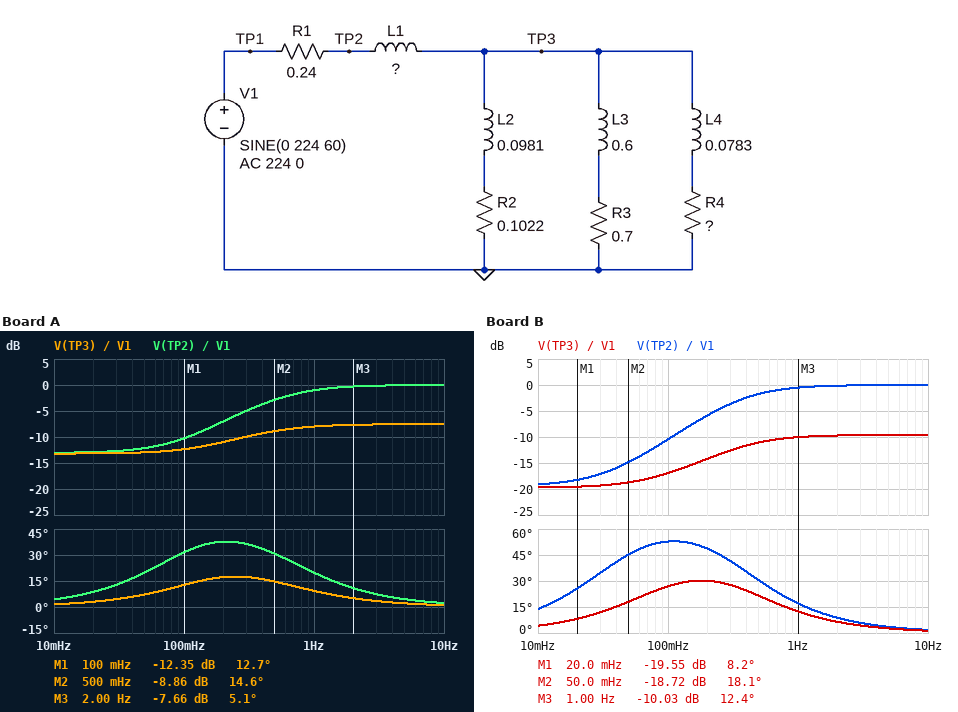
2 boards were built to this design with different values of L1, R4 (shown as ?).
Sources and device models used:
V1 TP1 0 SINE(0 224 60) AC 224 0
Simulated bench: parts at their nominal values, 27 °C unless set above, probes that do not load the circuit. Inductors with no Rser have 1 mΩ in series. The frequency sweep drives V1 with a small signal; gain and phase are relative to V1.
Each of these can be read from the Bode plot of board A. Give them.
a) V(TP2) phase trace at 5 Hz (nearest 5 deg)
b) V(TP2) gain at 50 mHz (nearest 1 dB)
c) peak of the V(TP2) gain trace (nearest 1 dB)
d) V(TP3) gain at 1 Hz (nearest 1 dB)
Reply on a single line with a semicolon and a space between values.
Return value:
5 deg; -12 dB; 0 dB; -8 dB
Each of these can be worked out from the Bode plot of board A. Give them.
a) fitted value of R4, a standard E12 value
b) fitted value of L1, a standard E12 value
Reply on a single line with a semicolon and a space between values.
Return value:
0.27 Ω; 56 mH
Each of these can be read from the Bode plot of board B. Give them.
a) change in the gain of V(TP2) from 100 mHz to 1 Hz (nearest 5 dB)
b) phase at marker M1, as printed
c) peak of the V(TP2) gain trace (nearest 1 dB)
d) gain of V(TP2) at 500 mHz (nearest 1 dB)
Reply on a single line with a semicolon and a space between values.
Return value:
10 dB; 8.2 deg; 0 dB; -2 dB
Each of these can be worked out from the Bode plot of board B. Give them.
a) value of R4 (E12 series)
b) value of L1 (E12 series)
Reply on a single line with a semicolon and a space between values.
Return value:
0.039 Ω; 82 mH
